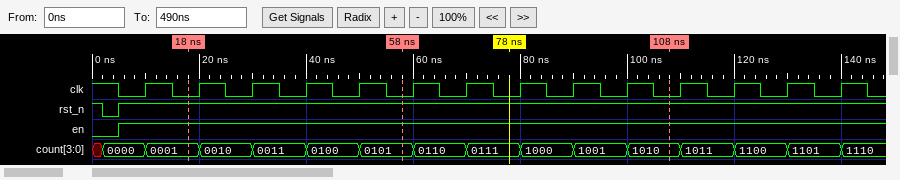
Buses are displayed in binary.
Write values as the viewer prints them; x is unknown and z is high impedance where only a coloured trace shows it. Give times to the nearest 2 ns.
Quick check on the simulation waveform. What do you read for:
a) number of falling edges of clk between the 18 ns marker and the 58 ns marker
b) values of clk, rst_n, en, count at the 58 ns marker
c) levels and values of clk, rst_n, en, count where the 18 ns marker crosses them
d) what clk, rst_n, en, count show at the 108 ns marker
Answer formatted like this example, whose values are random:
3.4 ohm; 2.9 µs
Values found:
4; clk=0, rst_n=1, en=1, count=0101; clk=0, rst_n=1, en=1, count=0001; clk=0, rst_n=1, en=1, count=1010
